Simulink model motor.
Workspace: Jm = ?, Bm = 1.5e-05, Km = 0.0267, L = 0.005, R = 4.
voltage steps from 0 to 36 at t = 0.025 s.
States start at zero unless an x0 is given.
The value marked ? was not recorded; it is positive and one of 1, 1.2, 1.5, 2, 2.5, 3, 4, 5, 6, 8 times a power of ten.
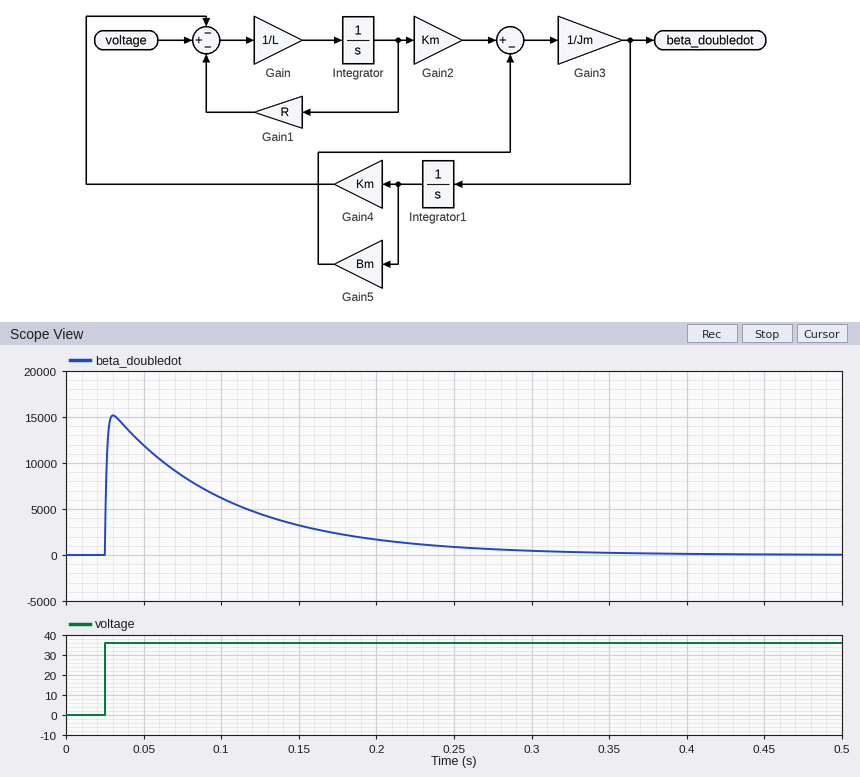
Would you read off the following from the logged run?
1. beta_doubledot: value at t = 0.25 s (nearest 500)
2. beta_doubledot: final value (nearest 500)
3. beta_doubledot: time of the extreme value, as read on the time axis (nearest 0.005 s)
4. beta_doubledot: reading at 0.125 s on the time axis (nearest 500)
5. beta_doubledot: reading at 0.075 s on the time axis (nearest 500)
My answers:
1000
0
0.030 s
4500
8500
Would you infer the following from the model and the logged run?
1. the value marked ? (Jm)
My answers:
1.5e-05
